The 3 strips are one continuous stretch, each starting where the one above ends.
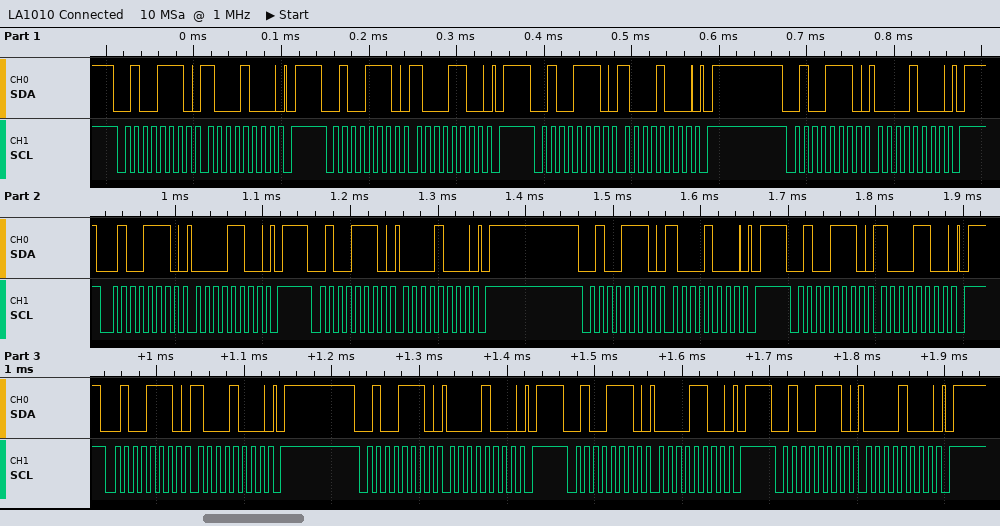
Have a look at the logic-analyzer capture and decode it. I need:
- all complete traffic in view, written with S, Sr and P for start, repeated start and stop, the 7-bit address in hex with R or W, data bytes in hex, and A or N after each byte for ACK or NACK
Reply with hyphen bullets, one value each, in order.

- S 27W A 88 A P S 27W A 8C A P S 27W A 88 A P S 27W A 08 A P S 27W A 0C A P S 27W A 08 A P S 27W A 88 A P S 27W A 8C A P S 27W A 88 A P S 27W A 08 A P S 27W A 0C A P S 27W A 08 A P
